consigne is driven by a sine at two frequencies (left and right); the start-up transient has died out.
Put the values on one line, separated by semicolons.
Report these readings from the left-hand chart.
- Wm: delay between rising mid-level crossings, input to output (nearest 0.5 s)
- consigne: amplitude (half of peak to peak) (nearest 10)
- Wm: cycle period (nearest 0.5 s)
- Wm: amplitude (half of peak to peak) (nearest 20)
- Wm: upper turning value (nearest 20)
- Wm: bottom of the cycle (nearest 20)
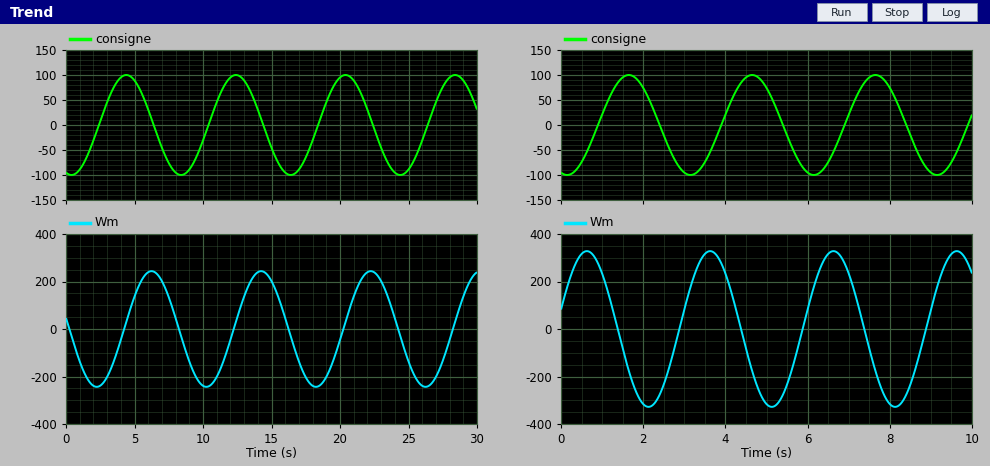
2.0 s; 100; 8.0 s; 240; 240; -240
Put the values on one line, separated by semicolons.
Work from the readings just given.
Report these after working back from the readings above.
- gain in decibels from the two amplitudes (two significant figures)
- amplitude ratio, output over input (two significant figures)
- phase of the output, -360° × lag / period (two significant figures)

7.6 dB; 2.4; -90°
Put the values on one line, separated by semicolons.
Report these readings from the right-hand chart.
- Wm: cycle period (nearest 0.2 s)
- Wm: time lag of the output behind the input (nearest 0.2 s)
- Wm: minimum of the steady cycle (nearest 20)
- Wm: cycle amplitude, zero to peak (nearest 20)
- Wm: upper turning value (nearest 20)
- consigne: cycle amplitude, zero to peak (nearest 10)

3.0 s; 2.0 s; -320; 320; 320; 100
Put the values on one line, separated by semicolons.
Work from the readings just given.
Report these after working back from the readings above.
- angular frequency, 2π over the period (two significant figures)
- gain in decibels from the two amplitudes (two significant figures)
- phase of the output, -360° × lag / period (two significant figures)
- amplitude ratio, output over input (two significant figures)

2.1 rad/s; 10 dB; -240°; 3.2
